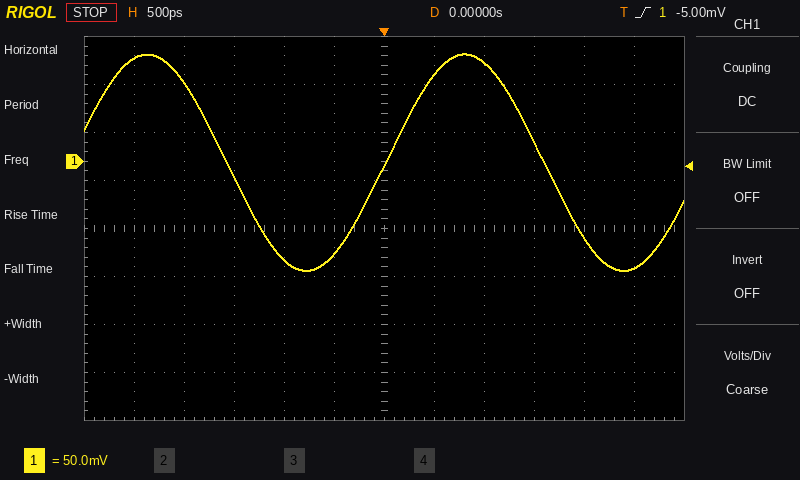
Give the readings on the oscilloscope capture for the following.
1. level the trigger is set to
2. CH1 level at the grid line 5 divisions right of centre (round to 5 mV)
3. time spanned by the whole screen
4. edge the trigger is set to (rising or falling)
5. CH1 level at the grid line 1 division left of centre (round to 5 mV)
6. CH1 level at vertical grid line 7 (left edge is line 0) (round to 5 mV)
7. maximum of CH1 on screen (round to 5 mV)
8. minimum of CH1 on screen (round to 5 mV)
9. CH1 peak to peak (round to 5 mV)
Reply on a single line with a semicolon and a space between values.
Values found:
-5.00 mV; -110 mV; 6 ns; rising; -95 mV; 90 mV; 110 mV; -115 mV; 225 mV
